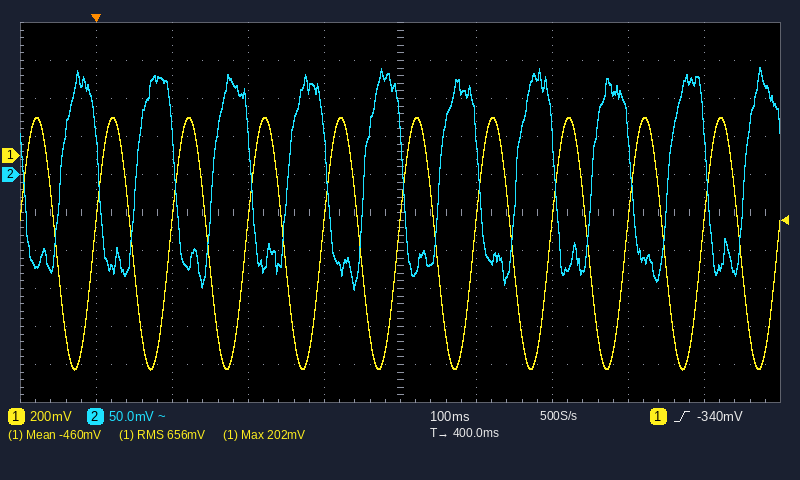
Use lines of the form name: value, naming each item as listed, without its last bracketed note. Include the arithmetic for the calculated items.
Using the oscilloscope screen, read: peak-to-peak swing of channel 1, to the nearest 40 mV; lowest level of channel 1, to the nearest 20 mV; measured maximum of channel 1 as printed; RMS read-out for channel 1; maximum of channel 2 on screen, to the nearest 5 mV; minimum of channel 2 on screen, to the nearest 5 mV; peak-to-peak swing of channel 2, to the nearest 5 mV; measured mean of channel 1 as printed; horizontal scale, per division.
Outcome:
peak-to-peak swing of channel 1, to the nearest 40 mV: 1.32 V
lowest level of channel 1, to the nearest 20 mV: -1.12 V
measured maximum of channel 1 as printed: 202 mV
RMS read-out for channel 1: 656 mV
maximum of channel 2 on screen, to the nearest 5 mV: 140 mV
minimum of channel 2 on screen, to the nearest 5 mV: -150 mV
peak-to-peak swing of channel 2, to the nearest 5 mV: 140 mV − (-150 mV) = 290 mV
measured mean of channel 1 as printed: -460 mV
horizontal scale, per division: 100 ms
